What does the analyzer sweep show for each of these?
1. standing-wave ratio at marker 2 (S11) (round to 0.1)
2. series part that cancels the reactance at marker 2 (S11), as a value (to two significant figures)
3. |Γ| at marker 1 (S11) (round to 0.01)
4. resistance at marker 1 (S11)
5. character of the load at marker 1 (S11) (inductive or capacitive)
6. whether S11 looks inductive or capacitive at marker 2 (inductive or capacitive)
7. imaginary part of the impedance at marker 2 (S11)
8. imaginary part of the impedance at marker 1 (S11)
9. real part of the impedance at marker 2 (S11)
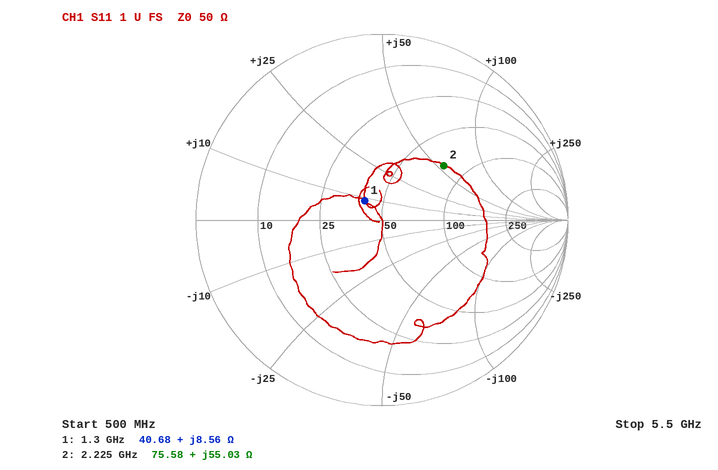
2.6
1.3 pF
0.14
40.68 Ω
inductive
inductive
+55.03 Ω
+8.56 Ω
75.58 Ω
